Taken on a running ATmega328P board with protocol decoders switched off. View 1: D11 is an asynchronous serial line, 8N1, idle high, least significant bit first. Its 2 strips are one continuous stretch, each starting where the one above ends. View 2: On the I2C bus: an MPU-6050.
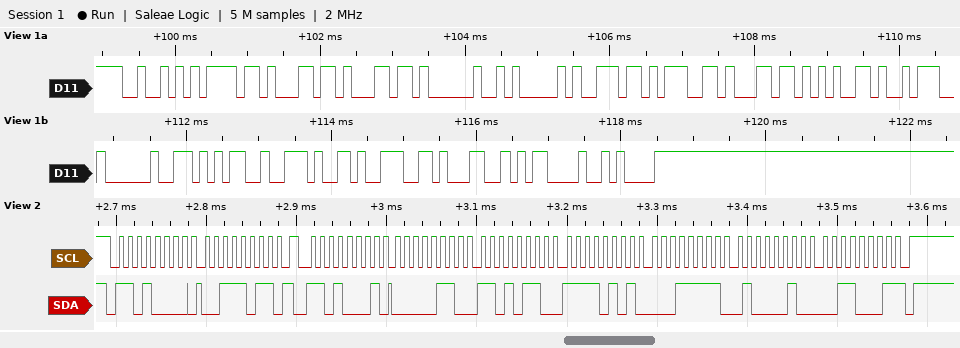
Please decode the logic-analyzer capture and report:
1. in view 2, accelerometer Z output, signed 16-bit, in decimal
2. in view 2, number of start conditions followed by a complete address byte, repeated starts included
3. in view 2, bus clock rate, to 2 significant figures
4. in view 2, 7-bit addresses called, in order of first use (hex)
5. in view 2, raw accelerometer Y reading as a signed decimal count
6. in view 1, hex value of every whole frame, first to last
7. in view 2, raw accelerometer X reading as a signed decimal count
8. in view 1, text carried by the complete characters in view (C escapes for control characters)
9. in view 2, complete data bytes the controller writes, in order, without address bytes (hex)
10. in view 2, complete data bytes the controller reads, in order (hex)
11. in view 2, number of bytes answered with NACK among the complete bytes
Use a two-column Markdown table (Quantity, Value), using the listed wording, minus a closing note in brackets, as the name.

| Quantity | Value |
|---|---|
| in view 2, accelerometer Z output, signed 16-bit, in decimal | 16945 |
| in view 2, number of start conditions followed by a complete address byte, repeated starts included | 2 |
| in view 2, bus clock rate, to 2 significant figures | 100 kHz |
| in view 2, 7-bit addresses called, in order of first use | 0x68 |
| in view 2, raw accelerometer Y reading as a signed decimal count | -2785 |
| in view 1, hex value of every whole frame, first to last | 52 6F 6C 6C 20 41 6E 67 6C 65 3A 20 35 2E 39 31 0D 0A |
| in view 2, raw accelerometer X reading as a signed decimal count | 1750 |
| in view 1, text carried by the complete characters in view | "Roll Angle: 5.91\r\n" |
| in view 2, complete data bytes the controller writes, in order, without address bytes | 3B |
| in view 2, complete data bytes the controller reads, in order | 06 D6 F5 1F 42 31 |
| in view 2, number of bytes answered with NACK among the complete bytes | 1 |
